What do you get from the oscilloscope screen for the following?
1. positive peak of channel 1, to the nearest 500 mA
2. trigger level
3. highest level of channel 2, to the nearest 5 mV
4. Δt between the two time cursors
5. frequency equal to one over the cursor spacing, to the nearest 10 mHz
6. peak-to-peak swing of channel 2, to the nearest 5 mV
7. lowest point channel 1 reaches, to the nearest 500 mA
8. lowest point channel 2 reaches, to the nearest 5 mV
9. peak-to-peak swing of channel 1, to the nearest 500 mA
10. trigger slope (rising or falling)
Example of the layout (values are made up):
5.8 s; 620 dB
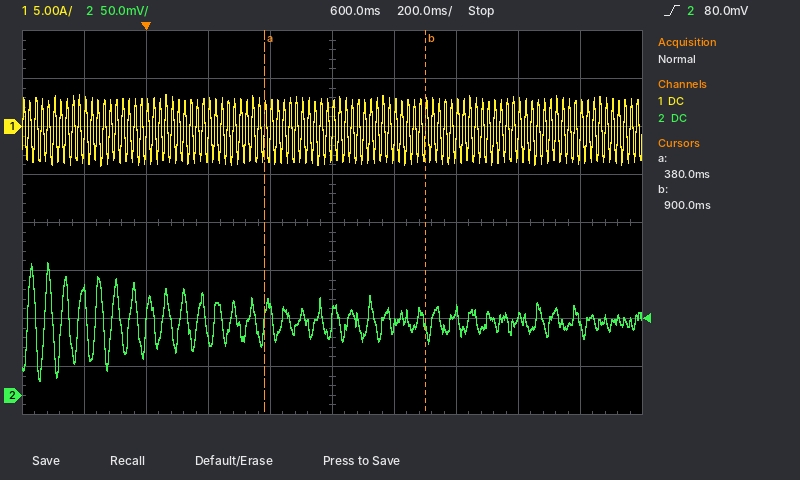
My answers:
3.5 A; 80.0 mV; 140 mV; 520 ms; 1.92 Hz; 125 mV; -4.0 A; 15 mV; 7.5 A; rising
